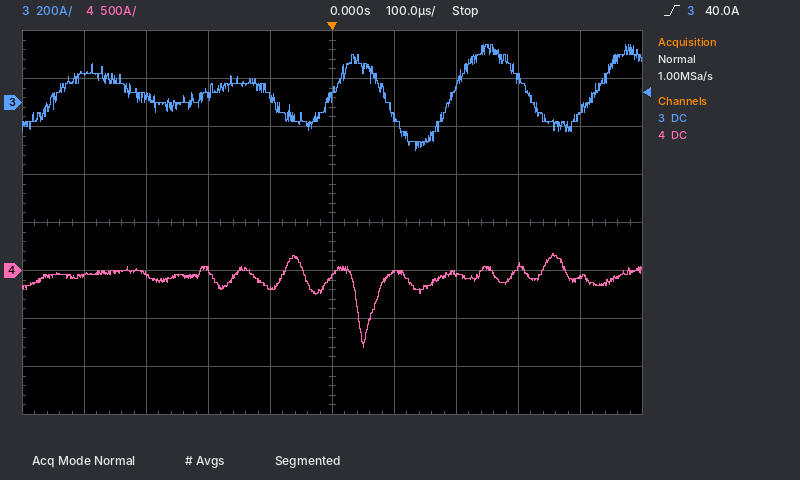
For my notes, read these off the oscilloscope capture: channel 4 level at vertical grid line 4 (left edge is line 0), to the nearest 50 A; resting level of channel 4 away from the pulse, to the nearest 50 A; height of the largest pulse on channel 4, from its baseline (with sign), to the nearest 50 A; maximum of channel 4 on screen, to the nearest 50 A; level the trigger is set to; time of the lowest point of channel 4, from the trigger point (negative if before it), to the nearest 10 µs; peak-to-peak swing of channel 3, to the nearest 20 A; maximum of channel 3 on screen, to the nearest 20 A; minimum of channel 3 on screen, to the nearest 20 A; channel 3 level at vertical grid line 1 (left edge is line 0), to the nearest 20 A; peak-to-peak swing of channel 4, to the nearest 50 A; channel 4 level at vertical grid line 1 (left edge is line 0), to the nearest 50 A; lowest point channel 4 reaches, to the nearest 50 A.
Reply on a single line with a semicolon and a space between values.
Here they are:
-200 A; -50 A; -750 A; 200 A; 40.0 A; +50 µs; 440 A; 240 A; -200 A; 120 A; 1.00 kA; -50 A; -800 A
